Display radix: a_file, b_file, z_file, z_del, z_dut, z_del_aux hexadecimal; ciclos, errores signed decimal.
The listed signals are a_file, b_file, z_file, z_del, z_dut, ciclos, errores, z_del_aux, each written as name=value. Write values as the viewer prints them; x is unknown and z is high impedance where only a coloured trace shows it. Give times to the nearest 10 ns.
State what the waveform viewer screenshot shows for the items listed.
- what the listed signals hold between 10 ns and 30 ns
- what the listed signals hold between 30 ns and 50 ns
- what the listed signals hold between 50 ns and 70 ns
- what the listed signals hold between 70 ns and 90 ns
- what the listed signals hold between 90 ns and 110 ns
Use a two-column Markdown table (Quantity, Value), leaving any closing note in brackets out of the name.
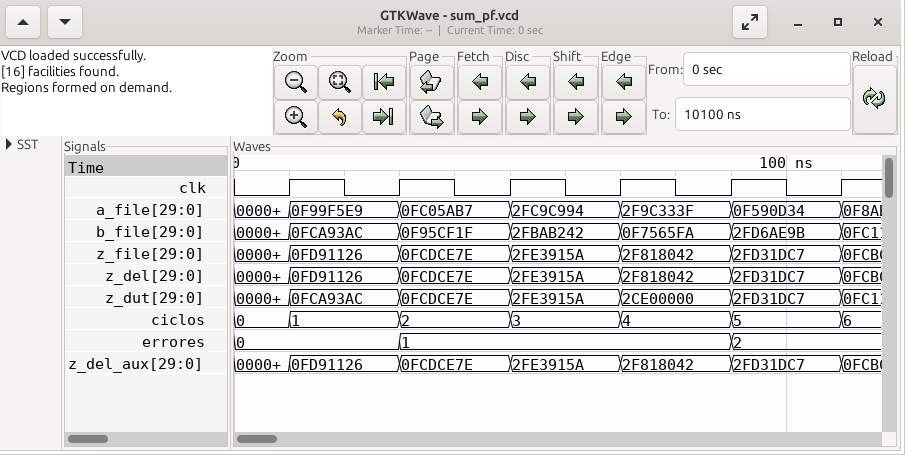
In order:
| Quantity | Value |
|---|---|
| what the listed signals hold between 10 ns and 30 ns | a_file=0F99F5E9, b_file=0FCA93AC, z_file=0FD91126, z_del=0FD91126, z_dut=0FCA93AC, ciclos=1, errores=0, z_del_aux=0FD91126 |
| what the listed signals hold between 30 ns and 50 ns | a_file=0FC05AB7, b_file=0F95CF1F, z_file=0FCDCE7E, z_del=0FCDCE7E, z_dut=0FCDCE7E, ciclos=2, errores=1, z_del_aux=0FCDCE7E |
| what the listed signals hold between 50 ns and 70 ns | a_file=2FC9C994, b_file=2FBAB242, z_file=2FE3915A, z_del=2FE3915A, z_dut=2FE3915A, ciclos=3, errores=1, z_del_aux=2FE3915A |
| what the listed signals hold between 70 ns and 90 ns | a_file=2F9C333F, b_file=0F7565FA, z_file=2F818042, z_del=2F818042, z_dut=2CE00000, ciclos=4, errores=1, z_del_aux=2F818042 |
| what the listed signals hold between 90 ns and 110 ns | a_file=0F590D34, b_file=2FD6AE9B, z_file=2FD31DC7, z_del=2FD31DC7, z_dut=2FD31DC7, ciclos=5, errores=2, z_del_aux=2FD31DC7 |
